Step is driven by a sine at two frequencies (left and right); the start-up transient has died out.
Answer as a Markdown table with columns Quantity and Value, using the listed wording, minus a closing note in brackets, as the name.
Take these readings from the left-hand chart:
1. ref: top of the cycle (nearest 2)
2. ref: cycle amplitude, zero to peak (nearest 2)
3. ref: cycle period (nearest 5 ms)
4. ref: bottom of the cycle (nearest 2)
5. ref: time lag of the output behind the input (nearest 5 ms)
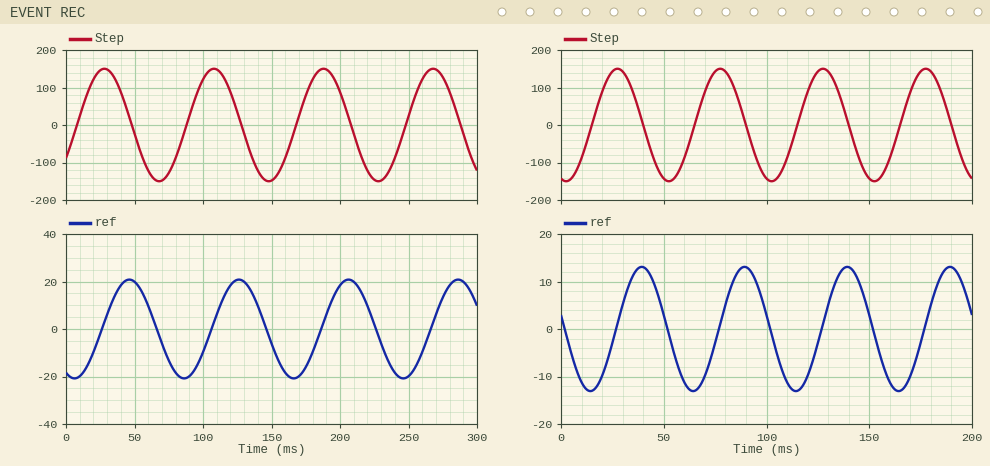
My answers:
| Quantity | Value |
|---|---|
| ref: top of the cycle | 20 |
| ref: cycle amplitude, zero to peak | 20 |
| ref: cycle period | 80 ms |
| ref: bottom of the cycle | -20 |
| ref: time lag of the output behind the input | 20 ms |
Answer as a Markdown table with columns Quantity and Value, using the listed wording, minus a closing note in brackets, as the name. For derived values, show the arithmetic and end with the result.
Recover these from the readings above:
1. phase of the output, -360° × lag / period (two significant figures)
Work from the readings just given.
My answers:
| Quantity | Value |
|---|---|
| phase of the output, -360° × lag / period | -360 × 20 / 80 = -90° |
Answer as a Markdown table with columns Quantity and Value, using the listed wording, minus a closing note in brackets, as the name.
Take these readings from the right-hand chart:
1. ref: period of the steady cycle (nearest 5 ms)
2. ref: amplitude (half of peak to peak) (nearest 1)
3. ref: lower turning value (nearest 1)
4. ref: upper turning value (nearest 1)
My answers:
| Quantity | Value |
|---|---|
| ref: period of the steady cycle | 50 ms |
| ref: amplitude (half of peak to peak) | 13 |
| ref: lower turning value | -13 |
| ref: upper turning value | 13 |
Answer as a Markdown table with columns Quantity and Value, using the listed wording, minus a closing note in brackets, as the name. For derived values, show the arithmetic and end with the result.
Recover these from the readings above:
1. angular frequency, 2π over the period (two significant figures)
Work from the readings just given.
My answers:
| Quantity | Value |
|---|---|
| angular frequency, 2π over the period | 2π / 50 = 0.13 rad/ms |
